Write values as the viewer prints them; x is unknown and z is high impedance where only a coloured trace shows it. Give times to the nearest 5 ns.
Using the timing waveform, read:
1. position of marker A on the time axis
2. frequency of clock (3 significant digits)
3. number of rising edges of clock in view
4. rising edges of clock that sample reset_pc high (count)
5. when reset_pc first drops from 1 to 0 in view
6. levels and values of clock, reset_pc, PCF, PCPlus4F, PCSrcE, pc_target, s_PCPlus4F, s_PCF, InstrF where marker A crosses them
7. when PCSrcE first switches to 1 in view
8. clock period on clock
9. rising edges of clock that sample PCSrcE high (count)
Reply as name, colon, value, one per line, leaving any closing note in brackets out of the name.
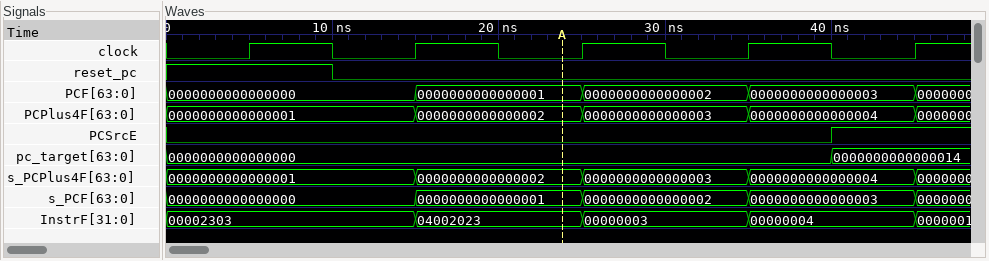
position of marker A on the time axis: 25 ns
frequency of clock: 100 MHz
number of rising edges of clock in view: 5
rising edges of clock that sample reset_pc high: 1
when reset_pc first drops from 1 to 0 in view: 10 ns
levels and values of clock, reset_pc, PCF, PCPlus4F, PCSrcE, pc_target, s_PCPlus4F, s_PCF, InstrF where marker A crosses them: clock=0, reset_pc=0, PCF=0000000000000001, PCPlus4F=0000000000000002, PCSrcE=0, pc_target=0000000000000000, s_PCPlus4F=0000000000000002, s_PCF=0000000000000001, InstrF=04002023
when PCSrcE first switches to 1 in view: 40 ns
clock period on clock: 10 ns
rising edges of clock that sample PCSrcE high: 1
